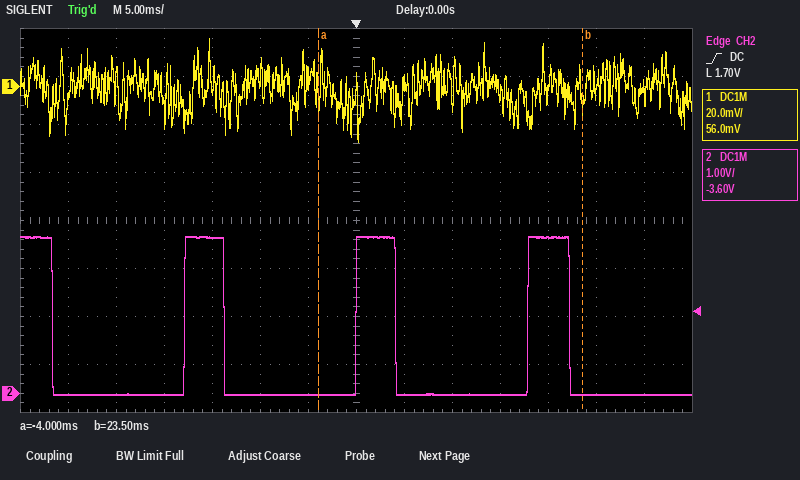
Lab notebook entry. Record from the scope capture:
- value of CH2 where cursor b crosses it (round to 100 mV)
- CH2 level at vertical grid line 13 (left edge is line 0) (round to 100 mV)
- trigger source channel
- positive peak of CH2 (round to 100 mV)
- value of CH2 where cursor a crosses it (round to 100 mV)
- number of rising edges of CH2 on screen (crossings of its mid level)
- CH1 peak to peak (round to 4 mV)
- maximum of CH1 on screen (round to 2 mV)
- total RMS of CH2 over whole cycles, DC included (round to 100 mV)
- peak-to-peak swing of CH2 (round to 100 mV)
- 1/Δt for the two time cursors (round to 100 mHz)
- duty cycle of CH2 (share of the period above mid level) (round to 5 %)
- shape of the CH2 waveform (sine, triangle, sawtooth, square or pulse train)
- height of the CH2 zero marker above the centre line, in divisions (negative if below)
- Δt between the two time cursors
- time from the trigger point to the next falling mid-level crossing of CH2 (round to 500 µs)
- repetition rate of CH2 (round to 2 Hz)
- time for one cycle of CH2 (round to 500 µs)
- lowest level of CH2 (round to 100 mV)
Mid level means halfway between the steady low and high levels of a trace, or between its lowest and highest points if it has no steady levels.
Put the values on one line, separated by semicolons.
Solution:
0.0 V; 0.0 V; CH2; 3.3 V; 0.0 V; 3; 44 mV; 20 mV; 1.6 V; 3.3 V; 36.4 Hz; 25 %; pulse train; -3.6 div; 27.5 ms; 4.0 ms; 56 Hz; 18.0 ms; 0.0 V
